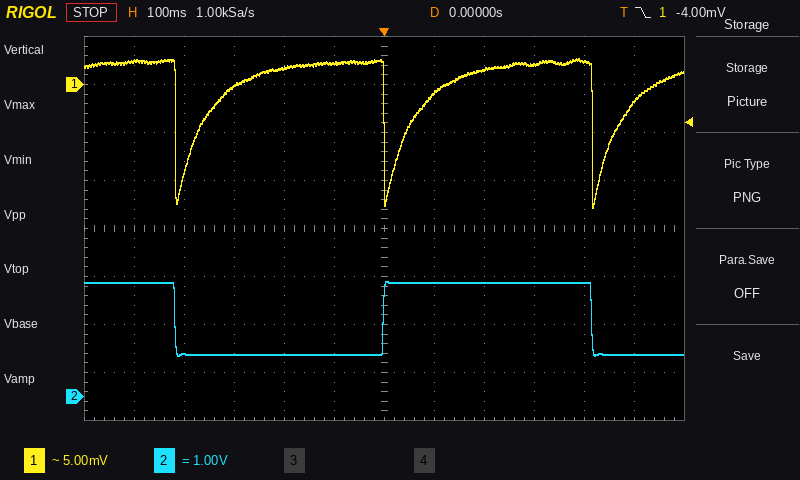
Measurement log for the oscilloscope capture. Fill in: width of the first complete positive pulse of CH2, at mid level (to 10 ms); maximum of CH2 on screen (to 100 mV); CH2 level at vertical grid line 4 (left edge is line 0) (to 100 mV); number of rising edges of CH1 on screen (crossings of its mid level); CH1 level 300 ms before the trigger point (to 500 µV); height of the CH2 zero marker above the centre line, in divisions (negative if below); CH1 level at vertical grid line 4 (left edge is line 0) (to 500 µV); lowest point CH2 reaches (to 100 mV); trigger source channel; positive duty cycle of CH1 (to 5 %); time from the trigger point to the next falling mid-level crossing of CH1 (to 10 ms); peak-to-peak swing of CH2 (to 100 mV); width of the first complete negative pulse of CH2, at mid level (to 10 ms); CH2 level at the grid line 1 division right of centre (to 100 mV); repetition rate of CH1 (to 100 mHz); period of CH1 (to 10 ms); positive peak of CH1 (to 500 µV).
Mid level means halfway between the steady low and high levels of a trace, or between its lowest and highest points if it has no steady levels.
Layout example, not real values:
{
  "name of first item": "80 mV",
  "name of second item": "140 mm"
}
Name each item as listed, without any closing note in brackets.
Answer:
{
  "width of the first complete positive pulse of CH2, at mid level": "420 ms",
  "maximum of CH2 on screen": "2.4 V",
  "CH2 level at vertical grid line 4 (left edge is line 0)": "900 mV",
  "number of rising edges of CH1 on screen": "3",
  "CH1 level 300 ms before the trigger point": "0.0 mV",
  "height of the CH2 zero marker above the centre line, in divisions": "-3.5 div",
  "CH1 level at vertical grid line 4 (left edge is line 0)": "1.5 mV",
  "lowest point CH2 reaches": "900 mV",
  "trigger source channel": "CH1",
  "positive duty cycle of CH1": "90 %",
  "time from the trigger point to the next falling mid-level crossing of CH1": "420 ms",
  "peak-to-peak swing of CH2": "1.5 V",
  "width of the first complete negative pulse of CH2, at mid level": "420 ms",
  "CH2 level at the grid line 1 division right of centre": "2.4 V",
  "repetition rate of CH1": "2.4 Hz",
  "period of CH1": "420 ms",
  "positive peak of CH1": "2.5 mV"
}
